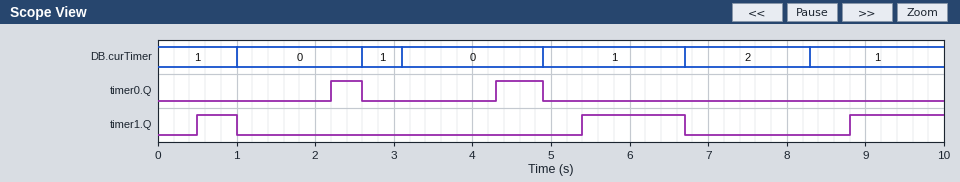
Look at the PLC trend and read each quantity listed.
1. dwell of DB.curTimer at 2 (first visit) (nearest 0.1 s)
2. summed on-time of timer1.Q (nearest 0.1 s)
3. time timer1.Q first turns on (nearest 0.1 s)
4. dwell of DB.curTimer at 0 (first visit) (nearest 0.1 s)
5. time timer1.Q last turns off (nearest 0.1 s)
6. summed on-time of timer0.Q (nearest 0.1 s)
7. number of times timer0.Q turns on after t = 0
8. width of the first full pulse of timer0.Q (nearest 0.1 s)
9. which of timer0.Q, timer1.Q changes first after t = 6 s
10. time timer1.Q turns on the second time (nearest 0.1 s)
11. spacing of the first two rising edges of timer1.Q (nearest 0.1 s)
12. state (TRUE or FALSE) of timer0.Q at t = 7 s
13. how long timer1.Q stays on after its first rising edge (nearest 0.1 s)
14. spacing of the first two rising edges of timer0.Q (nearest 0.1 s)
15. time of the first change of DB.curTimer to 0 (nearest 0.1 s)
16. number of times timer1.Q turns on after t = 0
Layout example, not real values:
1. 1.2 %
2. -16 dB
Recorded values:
1. 1.6 s
2. 3.0 s
3. 0.5 s
4. 1.6 s
5. 6.7 s
6. 1.0 s
7. 2
8. 0.4 s
9. timer1.Q
10. 5.4 s
11. 4.9 s
12. FALSE
13. 0.5 s
14. 2.1 s
15. 1.0 s
16. 3
